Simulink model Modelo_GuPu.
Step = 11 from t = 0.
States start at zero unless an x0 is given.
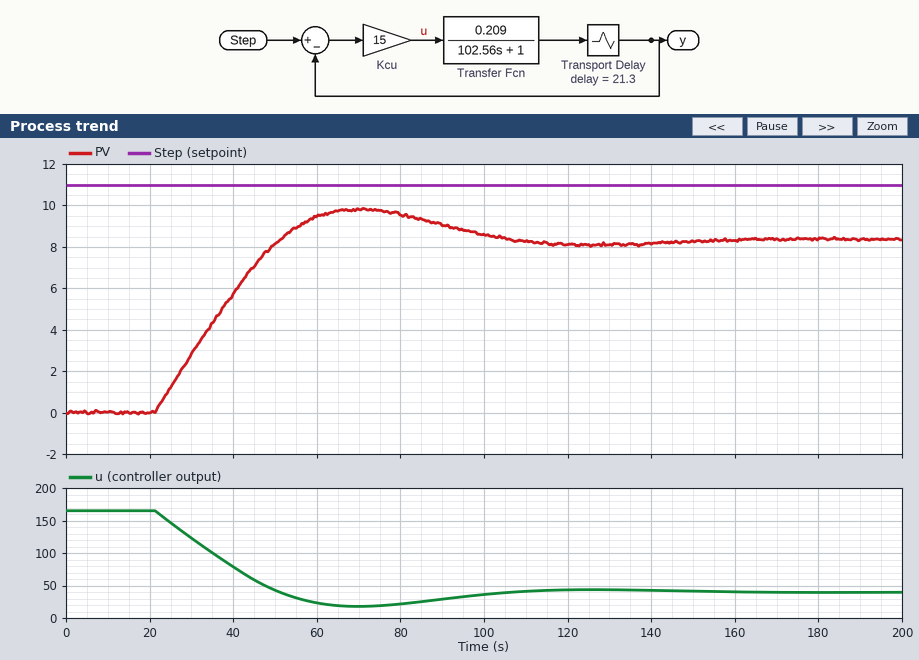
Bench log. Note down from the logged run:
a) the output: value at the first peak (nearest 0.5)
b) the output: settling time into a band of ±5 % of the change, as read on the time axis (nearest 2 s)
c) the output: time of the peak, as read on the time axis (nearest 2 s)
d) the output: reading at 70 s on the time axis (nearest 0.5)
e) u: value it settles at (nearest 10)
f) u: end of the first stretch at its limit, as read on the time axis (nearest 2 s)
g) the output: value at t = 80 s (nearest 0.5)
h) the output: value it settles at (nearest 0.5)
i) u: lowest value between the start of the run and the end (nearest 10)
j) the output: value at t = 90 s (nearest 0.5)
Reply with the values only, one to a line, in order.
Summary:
10.0
96 s
70 s
10.0
40
22 s
9.5
8.5
20
9.0
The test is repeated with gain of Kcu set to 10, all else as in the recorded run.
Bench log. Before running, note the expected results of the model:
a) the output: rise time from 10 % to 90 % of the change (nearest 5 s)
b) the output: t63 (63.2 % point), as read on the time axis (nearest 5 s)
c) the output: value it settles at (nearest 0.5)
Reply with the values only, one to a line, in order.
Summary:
35 s
45 s
7.5
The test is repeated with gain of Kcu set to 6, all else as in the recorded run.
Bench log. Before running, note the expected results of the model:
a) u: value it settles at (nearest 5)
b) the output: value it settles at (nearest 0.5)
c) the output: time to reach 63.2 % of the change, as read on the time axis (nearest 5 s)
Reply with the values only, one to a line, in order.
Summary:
30
6.0
55 s
